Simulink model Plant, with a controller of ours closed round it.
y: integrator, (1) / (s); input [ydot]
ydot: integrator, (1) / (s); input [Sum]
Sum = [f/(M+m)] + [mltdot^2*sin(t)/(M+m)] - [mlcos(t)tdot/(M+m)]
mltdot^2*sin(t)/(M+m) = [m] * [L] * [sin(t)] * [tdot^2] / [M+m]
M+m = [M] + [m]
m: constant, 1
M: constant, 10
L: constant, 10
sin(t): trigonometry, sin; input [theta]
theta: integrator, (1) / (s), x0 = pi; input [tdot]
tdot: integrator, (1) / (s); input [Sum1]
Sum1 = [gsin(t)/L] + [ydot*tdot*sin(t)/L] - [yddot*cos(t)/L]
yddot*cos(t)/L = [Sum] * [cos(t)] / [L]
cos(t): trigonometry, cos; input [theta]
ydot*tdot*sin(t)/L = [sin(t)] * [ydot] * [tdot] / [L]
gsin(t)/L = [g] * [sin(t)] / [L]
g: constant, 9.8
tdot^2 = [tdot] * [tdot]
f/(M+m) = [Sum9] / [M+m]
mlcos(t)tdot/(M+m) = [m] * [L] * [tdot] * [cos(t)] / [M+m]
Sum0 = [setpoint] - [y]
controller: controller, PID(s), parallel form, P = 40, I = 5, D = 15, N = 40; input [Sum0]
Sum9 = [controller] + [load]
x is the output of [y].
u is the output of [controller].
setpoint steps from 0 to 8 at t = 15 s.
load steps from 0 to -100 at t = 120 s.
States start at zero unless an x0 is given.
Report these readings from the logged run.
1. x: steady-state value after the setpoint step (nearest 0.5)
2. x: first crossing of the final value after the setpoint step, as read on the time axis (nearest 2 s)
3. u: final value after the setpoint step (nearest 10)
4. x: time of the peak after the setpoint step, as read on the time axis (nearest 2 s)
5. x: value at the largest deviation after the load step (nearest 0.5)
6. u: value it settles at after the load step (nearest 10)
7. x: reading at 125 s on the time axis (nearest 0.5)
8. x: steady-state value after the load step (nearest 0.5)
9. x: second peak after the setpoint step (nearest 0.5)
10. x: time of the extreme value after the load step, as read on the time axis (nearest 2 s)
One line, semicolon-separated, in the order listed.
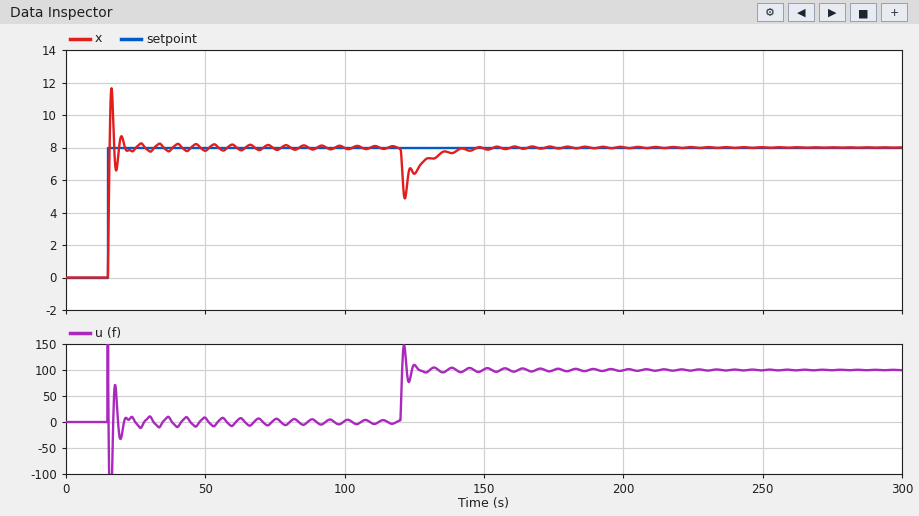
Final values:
8.0; 16 s; 0; 16 s; 5.0; 100; 6.5; 8.0; 8.5; 122 s
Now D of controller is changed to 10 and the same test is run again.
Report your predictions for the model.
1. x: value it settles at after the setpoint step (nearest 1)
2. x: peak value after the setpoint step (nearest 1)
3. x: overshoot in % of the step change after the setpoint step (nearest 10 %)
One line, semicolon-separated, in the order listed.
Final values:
8; 13; 60 %
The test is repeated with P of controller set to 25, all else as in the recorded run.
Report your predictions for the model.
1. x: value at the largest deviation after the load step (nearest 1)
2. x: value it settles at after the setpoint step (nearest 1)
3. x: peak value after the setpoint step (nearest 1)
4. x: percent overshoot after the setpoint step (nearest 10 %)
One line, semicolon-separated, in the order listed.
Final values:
4; 8; 11; 40 %
